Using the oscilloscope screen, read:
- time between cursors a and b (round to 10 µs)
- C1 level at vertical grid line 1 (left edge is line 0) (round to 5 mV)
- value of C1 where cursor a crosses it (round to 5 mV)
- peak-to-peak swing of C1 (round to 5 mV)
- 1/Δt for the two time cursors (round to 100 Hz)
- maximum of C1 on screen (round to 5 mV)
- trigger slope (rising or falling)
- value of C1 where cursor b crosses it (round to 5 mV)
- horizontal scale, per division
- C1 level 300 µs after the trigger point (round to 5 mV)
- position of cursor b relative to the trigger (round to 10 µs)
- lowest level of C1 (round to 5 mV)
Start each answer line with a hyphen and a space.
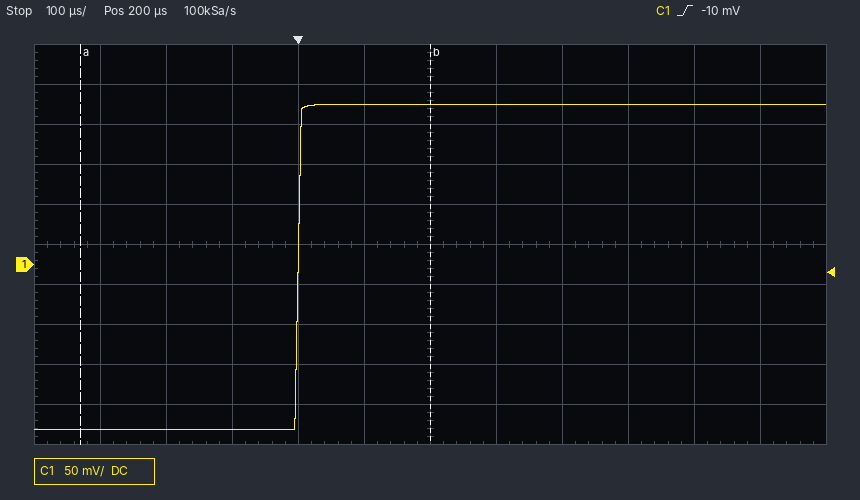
- 530 µs
- -205 mV
- -205 mV
- 405 mV
- 1.9 kHz
- 200 mV
- rising
- 200 mV
- 100 µs
- 200 mV
- +200 µs
- -205 mV
